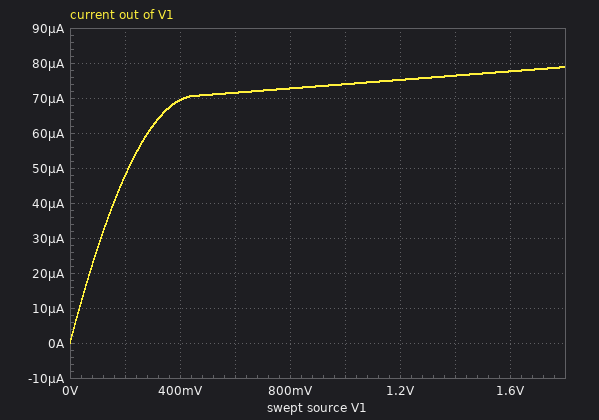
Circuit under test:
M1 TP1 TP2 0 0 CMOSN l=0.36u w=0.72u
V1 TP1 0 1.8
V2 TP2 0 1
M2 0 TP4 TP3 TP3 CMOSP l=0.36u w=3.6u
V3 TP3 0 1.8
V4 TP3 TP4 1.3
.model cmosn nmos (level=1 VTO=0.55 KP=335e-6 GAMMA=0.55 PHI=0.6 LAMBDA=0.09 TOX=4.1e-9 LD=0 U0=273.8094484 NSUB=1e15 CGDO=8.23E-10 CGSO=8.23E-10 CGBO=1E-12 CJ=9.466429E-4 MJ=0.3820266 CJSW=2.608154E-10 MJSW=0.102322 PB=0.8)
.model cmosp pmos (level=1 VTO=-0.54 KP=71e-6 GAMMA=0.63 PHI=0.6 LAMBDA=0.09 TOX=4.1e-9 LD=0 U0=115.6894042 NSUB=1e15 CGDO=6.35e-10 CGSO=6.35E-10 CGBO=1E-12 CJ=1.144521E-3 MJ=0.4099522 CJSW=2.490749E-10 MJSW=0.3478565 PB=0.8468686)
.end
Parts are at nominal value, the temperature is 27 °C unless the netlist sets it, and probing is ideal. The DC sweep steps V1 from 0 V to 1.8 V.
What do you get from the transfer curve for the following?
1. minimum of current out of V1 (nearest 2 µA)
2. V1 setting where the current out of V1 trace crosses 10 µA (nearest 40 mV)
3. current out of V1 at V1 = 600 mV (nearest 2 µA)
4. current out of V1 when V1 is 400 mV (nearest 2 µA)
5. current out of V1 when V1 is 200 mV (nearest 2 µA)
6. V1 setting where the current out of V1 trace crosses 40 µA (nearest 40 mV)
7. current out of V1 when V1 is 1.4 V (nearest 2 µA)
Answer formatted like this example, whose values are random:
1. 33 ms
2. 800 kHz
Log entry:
1. 0 A
2. 40 mV
3. 72 µA
4. 70 µA
5. 48 µA
6. 160 mV
7. 76 µA
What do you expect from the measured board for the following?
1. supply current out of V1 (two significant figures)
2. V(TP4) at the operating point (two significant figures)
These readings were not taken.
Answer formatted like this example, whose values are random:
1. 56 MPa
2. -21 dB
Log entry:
1. 79 µA
2. 500 mV
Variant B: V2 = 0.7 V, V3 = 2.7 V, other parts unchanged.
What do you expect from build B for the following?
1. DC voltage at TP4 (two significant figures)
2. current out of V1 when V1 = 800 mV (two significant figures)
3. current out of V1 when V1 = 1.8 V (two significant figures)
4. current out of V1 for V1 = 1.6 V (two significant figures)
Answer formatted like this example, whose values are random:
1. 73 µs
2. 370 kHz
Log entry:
1. 1.4 V
2. 8.1 µA
3. 8.8 µA
4. 8.6 µA
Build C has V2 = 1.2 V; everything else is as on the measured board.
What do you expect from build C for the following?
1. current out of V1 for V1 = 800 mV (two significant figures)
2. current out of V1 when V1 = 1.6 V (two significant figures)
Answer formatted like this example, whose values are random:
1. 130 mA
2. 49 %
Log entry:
1. 150 µA
2. 160 µA
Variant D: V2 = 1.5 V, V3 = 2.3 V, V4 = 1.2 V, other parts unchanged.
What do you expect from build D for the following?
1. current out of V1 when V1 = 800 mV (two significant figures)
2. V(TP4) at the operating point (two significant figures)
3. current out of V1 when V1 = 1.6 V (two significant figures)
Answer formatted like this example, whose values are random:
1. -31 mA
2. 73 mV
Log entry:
1. 320 µA
2. 1.1 V
3. 350 µA
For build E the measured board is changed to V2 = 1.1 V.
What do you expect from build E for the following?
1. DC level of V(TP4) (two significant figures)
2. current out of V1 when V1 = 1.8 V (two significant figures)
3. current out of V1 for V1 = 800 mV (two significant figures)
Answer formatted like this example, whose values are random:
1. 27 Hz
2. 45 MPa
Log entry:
1. 500 mV
2. 120 µA
3. 110 µA
